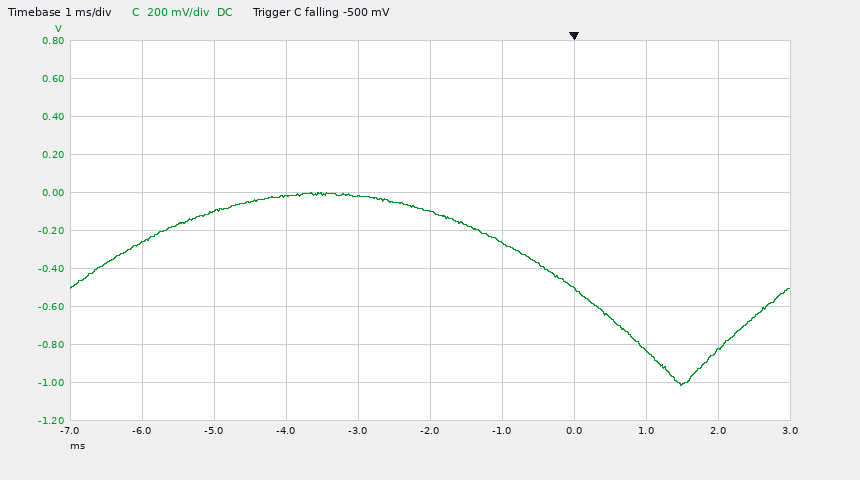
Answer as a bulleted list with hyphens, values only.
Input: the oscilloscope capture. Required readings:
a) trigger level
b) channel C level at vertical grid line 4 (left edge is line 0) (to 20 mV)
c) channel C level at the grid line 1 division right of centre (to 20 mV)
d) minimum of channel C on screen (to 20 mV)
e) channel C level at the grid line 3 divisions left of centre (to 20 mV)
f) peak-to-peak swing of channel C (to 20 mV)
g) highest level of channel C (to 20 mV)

- -500 mV
- -20 mV
- -260 mV
- -1.02 V
- -100 mV
- 1.02 V
- 0 mV
